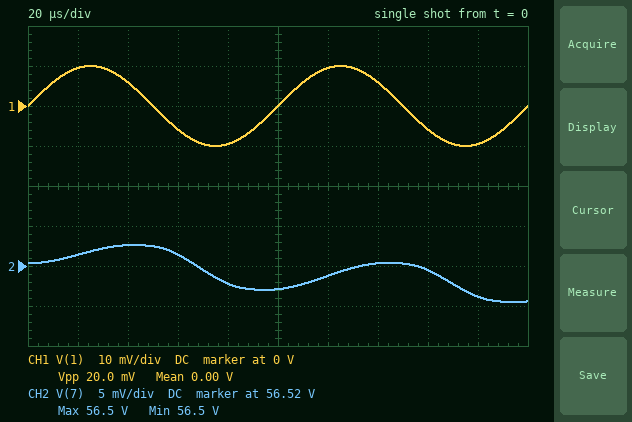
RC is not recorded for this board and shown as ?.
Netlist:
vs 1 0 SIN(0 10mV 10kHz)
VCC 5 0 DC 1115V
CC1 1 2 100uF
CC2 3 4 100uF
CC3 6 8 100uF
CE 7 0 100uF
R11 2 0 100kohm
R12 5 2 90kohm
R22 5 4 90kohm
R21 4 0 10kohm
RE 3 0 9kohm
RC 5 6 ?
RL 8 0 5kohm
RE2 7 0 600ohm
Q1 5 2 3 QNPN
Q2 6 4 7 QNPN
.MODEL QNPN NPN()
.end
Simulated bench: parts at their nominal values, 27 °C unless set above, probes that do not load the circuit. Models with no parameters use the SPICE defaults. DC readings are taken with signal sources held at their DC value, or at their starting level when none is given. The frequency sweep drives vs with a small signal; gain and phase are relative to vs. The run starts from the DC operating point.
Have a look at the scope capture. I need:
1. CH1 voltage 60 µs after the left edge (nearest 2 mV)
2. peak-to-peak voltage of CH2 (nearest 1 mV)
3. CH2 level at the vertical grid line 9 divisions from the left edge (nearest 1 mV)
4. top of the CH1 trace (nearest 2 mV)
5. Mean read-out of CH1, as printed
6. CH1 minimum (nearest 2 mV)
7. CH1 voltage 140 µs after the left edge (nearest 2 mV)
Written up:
-6 mV
7 mV
56.521 V
10 mV
0.00 V
-10 mV
6 mV
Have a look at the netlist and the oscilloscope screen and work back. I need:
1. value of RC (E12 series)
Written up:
12 kΩ
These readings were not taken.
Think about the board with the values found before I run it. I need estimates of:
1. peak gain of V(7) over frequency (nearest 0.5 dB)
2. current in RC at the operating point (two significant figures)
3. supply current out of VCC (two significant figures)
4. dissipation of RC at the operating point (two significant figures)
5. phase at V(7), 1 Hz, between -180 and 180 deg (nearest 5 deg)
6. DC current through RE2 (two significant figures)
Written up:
-6.0 dB
88 mA
170 mA
93 W
60 deg
94 mA
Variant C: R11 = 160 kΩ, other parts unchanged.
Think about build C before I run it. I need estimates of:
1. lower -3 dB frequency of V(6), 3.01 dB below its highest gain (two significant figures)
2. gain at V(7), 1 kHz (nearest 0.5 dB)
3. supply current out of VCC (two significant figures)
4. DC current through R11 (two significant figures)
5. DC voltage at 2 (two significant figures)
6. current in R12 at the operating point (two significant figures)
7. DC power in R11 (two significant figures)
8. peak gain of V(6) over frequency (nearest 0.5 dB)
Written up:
3.7 kHz
-6.5 dB
180 mA
4.2 mA
670 V
4.9 mA
2.8 W
14.5 dB
